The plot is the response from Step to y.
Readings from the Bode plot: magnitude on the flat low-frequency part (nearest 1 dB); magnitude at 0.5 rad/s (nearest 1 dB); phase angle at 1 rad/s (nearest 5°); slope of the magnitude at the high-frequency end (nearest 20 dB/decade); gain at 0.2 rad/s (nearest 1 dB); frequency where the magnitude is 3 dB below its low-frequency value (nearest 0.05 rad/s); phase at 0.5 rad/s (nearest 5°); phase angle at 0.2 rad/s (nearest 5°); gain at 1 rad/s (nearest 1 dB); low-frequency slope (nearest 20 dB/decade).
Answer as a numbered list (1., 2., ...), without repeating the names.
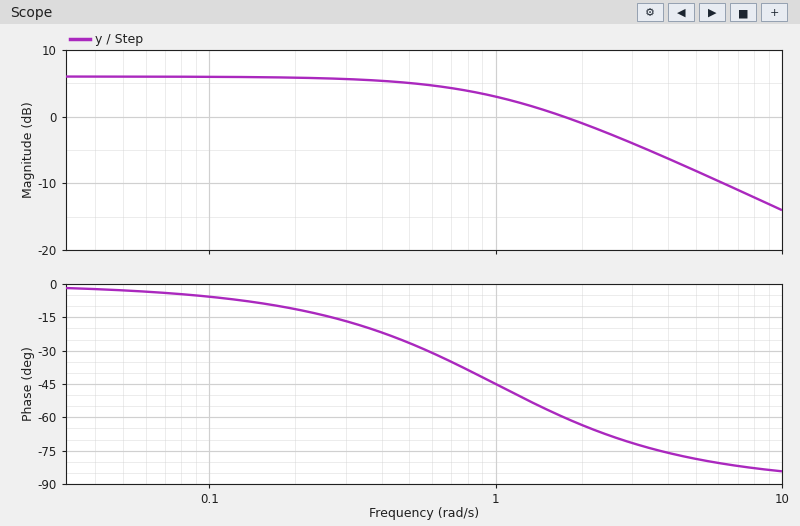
1. 6 dB
2. 5 dB
3. -45°
4. -20 dB/decade
5. 6 dB
6. 1.00 rad/s
7. -25°
8. -10°
9. 3 dB
10. 0 dB/decade
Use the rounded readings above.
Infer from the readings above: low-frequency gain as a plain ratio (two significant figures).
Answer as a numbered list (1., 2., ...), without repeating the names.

1. 2.0
